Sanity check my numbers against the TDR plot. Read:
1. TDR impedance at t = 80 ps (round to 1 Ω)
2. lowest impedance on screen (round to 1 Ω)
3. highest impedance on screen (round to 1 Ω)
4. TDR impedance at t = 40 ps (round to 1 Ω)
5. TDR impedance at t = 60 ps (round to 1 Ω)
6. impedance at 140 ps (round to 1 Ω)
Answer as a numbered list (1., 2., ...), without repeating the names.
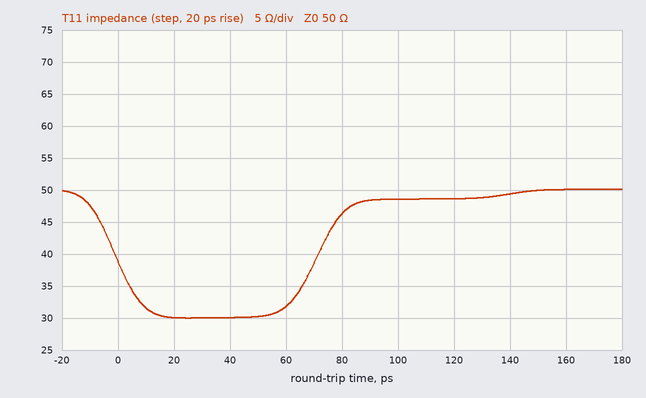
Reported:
1. 46 Ω
2. 30 Ω
3. 50 Ω
4. 30 Ω
5. 32 Ω
6. 49 Ω
